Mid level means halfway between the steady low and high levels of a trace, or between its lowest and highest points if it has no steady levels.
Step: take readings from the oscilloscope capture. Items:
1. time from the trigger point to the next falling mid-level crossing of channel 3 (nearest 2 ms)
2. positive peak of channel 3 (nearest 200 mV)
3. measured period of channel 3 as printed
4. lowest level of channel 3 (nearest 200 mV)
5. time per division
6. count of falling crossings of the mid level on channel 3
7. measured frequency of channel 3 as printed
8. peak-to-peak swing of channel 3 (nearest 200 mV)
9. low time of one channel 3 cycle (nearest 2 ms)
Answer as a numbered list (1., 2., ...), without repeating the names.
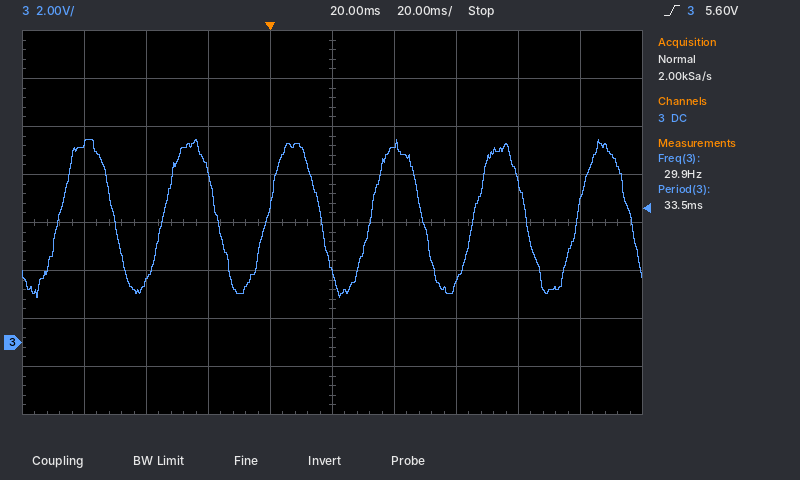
1. 16 ms
2. 8.4 V
3. 33.5 ms
4. 1.8 V
5. 20 ms
6. 6
7. 29.9 Hz
8. 6.6 V
9. 16 ms
